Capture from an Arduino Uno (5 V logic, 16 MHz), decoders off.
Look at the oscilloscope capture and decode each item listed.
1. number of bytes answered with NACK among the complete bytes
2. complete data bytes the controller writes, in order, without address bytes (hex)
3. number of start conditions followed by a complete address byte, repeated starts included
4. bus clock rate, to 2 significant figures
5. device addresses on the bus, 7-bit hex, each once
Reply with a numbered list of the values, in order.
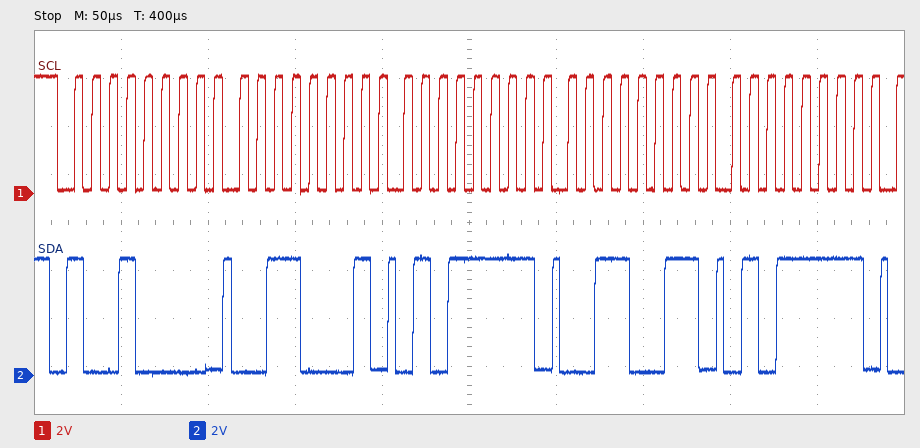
1. 0
2. 31 5F 33 5F
3. 1
4. 100 kHz
5. 0x48
